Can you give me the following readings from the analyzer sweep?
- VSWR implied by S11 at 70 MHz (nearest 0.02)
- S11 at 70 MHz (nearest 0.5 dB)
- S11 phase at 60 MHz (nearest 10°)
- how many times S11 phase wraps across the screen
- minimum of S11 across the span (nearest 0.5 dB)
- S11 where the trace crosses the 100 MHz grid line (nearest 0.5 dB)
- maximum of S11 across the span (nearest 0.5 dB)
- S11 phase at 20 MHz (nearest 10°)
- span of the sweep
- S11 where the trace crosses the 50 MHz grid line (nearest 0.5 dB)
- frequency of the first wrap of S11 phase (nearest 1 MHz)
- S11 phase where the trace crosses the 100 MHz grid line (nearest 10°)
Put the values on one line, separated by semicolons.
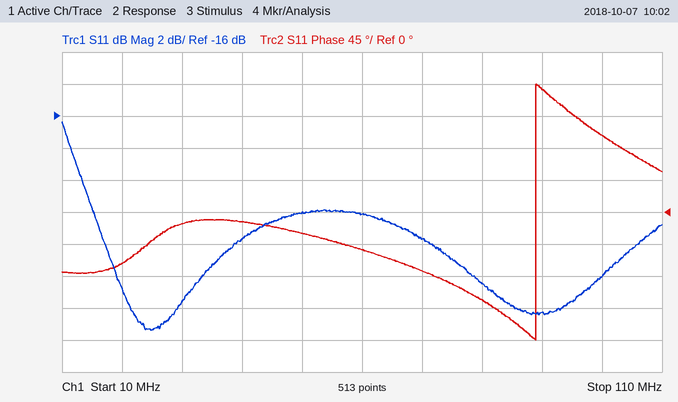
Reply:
1.14; -23.5 dB; -50°; 1; -29.5 dB; -26.0 dB; -16.5 dB; -70°; 100 MHz; -22.0 dB; 89 MHz; 110°
